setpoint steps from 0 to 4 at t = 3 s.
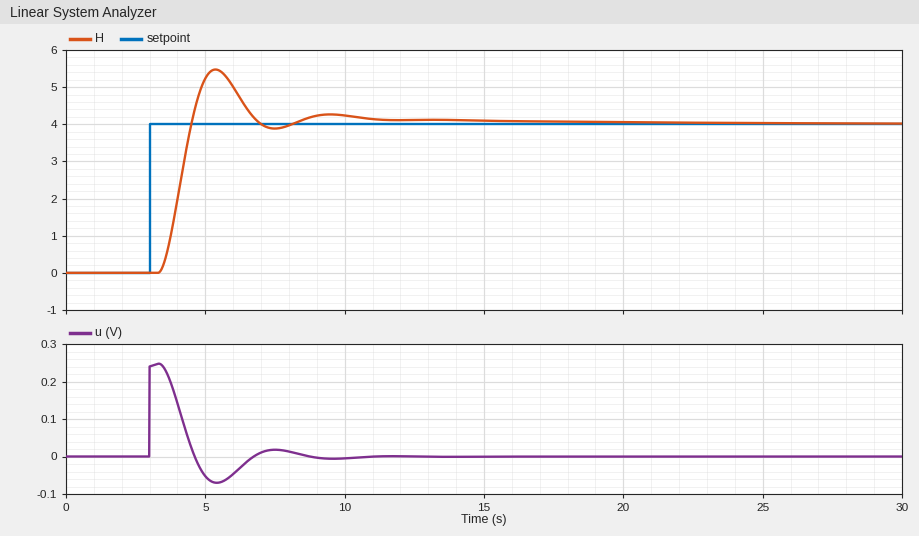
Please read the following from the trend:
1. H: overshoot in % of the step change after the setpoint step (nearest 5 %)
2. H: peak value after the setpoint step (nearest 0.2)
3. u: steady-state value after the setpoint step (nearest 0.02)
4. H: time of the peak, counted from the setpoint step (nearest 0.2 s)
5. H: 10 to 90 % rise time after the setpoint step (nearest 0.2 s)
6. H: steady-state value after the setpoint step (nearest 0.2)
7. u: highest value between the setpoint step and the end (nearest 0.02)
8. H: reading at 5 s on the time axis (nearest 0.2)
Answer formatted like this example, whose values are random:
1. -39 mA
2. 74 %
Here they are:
1. 35 %
2. 5.4
3. 0.00
4. 2.4 s
5. 0.8 s
6. 4.0
7. 0.24
8. 5.2
